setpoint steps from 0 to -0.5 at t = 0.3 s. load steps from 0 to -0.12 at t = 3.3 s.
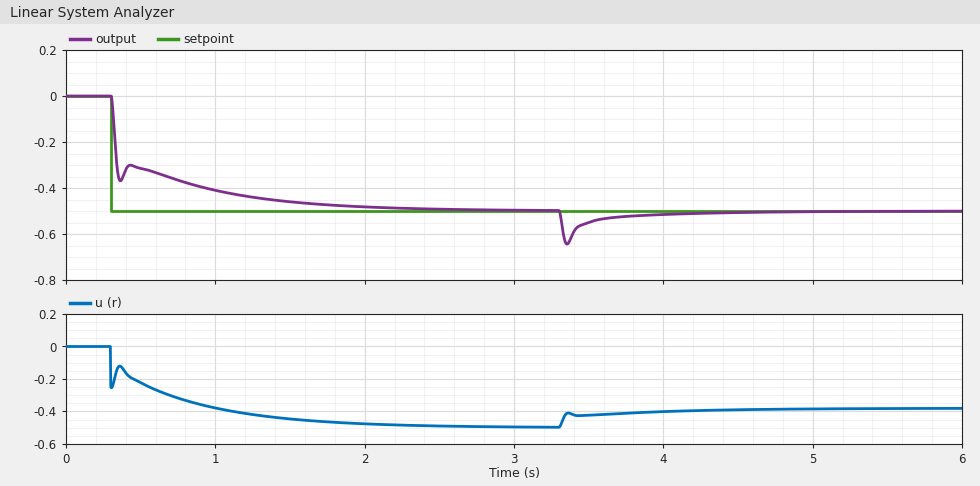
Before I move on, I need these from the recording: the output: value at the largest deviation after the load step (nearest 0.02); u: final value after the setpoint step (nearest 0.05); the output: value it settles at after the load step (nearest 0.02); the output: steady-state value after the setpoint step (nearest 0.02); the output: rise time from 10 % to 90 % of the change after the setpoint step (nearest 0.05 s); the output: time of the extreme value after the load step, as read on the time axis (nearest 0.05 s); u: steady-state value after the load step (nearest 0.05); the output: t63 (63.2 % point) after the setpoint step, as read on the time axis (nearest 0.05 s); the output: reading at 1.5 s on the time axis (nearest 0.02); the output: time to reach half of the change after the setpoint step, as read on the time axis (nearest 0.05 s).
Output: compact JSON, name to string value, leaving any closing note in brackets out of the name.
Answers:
{"the output: value at the largest deviation after the load step": "-0.64", "u: final value after the setpoint step": "-0.50", "the output: value it settles at after the load step": "-0.50", "the output: steady-state value after the setpoint step": "-0.50", "the output: rise time from 10 % to 90 % of the change after the setpoint step": "1.05 s", "the output: time of the extreme value after the load step, as read on the time axis": "3.35 s", "u: steady-state value after the load step": "-0.40", "the output: t63 (63.2 % point) after the setpoint step, as read on the time axis": "0.35 s", "the output: reading at 1.5 s on the time axis": "-0.46", "the output: time to reach half of the change after the setpoint step, as read on the time axis": "0.35 s"}
